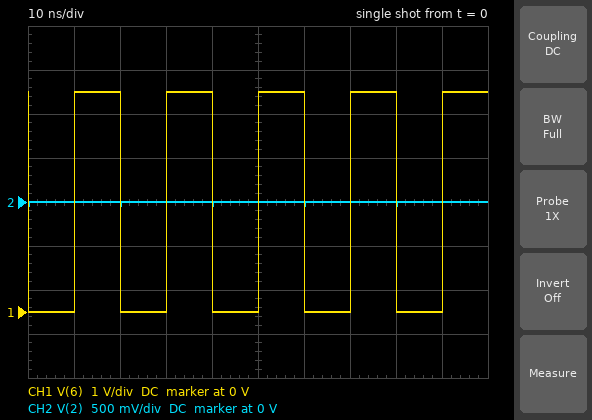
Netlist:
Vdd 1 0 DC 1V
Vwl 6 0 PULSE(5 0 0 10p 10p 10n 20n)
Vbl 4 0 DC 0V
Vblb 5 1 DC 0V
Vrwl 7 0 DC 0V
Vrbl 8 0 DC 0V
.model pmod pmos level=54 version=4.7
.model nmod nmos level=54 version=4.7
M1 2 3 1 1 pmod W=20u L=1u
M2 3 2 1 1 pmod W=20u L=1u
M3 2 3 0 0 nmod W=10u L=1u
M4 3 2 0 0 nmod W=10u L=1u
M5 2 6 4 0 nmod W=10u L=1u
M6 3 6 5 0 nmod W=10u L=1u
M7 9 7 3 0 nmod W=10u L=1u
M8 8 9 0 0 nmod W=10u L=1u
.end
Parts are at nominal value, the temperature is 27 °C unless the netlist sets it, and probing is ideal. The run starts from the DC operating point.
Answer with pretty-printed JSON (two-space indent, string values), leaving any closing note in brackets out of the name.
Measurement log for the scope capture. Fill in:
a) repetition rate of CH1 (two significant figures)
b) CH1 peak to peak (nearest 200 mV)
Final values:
{
  "repetition rate of CH1": "50 MHz",
  "CH1 peak to peak": "5.0 V"
}
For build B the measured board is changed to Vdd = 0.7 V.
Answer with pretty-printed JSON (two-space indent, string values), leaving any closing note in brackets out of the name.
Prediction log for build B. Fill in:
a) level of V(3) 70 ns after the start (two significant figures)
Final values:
{
  "level of V(3) 70 ns after the start": "700 mV"
}
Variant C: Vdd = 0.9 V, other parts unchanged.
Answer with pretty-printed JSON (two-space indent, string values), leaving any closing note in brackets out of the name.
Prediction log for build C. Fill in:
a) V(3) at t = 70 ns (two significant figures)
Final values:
{
  "V(3) at t = 70 ns": "900 mV"
}
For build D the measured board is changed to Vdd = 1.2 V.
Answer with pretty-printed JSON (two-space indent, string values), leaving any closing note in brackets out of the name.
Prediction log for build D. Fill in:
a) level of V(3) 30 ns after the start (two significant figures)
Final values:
{
  "level of V(3) 30 ns after the start": "1.2 V"
}
